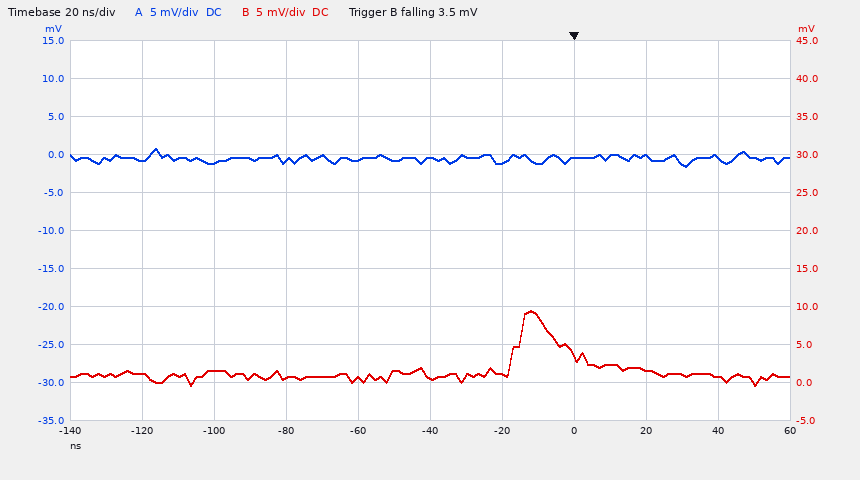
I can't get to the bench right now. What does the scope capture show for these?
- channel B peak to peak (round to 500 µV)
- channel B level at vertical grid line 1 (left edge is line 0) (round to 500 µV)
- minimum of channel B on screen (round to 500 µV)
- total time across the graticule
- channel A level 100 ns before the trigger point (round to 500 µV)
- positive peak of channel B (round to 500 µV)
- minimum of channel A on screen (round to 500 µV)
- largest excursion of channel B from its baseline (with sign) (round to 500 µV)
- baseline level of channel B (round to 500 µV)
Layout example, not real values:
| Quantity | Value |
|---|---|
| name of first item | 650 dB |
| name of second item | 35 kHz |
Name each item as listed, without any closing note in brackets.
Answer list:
| Quantity | Value |
|---|---|
| channel B peak to peak | 10.0 mV |
| channel B level at vertical grid line 1 (left edge is line 0) | 1.0 mV |
| minimum of channel B on screen | -500 µV |
| total time across the graticule | 200 ns |
| channel A level 100 ns before the trigger point | -1.0 mV |
| positive peak of channel B | 9.5 mV |
| minimum of channel A on screen | -1.5 mV |
| largest excursion of channel B from its baseline (with sign) | +8.5 mV |
| baseline level of channel B | 1.0 mV |
